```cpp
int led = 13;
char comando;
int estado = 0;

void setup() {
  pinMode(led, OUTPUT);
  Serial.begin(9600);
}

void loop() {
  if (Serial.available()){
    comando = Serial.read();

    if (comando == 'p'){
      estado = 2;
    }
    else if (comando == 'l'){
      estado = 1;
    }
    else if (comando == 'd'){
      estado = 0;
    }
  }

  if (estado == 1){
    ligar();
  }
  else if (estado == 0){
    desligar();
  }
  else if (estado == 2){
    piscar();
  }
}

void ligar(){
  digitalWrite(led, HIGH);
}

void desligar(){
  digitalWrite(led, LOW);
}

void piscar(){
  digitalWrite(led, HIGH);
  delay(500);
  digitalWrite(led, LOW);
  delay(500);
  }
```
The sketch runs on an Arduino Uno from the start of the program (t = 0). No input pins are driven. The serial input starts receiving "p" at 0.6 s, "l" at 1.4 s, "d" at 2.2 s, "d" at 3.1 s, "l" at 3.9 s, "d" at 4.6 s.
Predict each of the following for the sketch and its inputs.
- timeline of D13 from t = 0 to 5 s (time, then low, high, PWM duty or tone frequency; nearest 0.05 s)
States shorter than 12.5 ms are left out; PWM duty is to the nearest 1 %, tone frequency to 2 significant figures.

0 s low; 0.6 s high; 1.1 s low; 1.6 s high; 2.2 s low; 3.9 s high; 4.6 s low
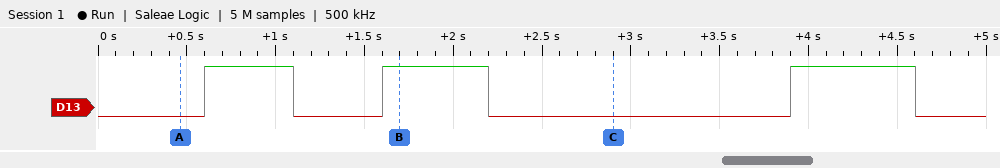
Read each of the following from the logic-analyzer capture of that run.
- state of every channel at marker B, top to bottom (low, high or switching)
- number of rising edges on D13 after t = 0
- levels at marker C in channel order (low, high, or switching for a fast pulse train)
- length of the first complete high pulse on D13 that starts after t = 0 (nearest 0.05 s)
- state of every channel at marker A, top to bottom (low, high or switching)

D13 high
3
D13 low
0.50 s
D13 low
